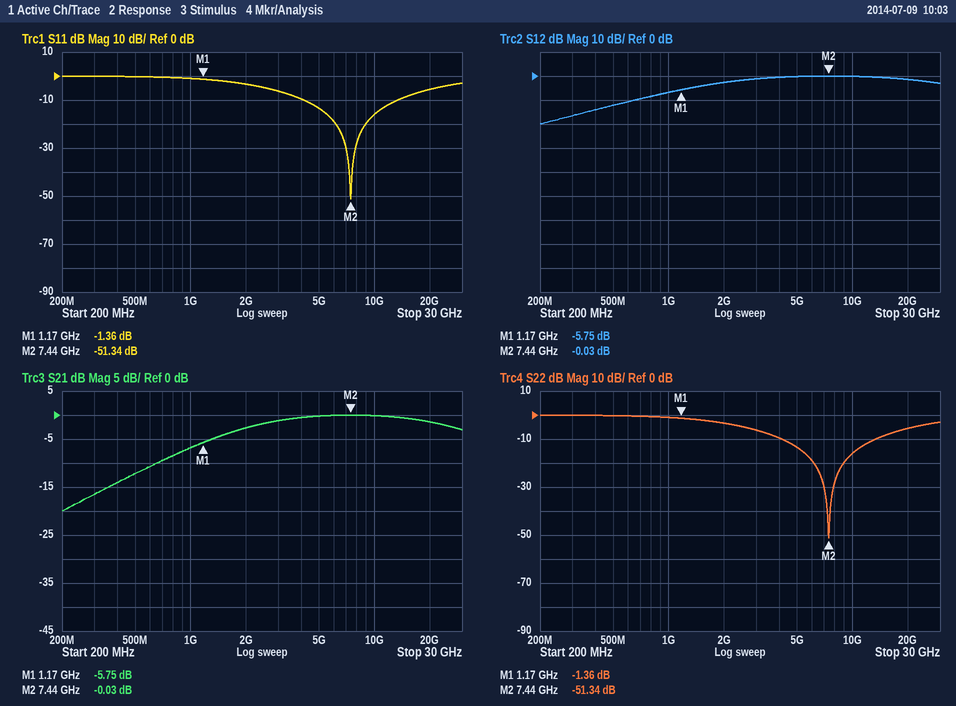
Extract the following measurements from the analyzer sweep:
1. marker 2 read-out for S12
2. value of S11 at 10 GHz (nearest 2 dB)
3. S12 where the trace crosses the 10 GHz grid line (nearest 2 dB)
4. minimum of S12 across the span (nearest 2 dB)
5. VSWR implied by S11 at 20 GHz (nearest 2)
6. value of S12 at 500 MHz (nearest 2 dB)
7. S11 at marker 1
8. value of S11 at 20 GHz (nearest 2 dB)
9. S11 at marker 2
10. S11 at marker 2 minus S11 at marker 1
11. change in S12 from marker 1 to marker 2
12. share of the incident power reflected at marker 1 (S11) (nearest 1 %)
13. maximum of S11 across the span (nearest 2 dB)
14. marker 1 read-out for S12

-0.03 dB
-16 dB
0 dB
-20 dB
4
-12 dB
-1.36 dB
-6 dB
-51.34 dB
-49.98 dB
5.72 dB
73 %
0 dB
-5.75 dB
